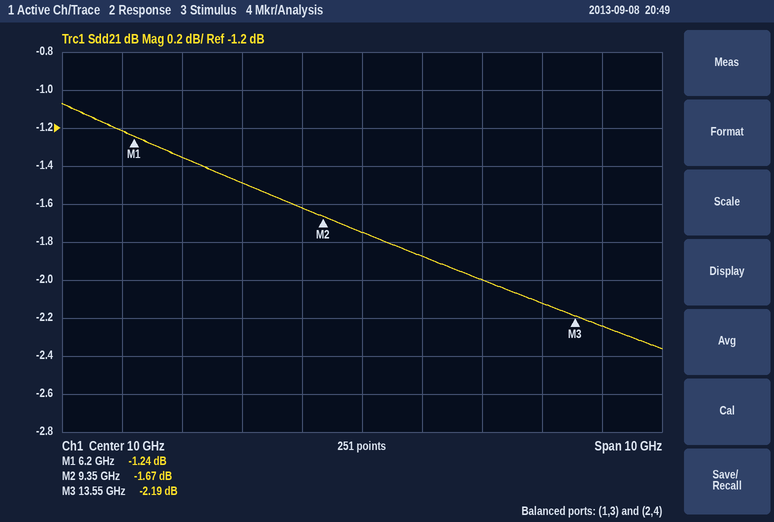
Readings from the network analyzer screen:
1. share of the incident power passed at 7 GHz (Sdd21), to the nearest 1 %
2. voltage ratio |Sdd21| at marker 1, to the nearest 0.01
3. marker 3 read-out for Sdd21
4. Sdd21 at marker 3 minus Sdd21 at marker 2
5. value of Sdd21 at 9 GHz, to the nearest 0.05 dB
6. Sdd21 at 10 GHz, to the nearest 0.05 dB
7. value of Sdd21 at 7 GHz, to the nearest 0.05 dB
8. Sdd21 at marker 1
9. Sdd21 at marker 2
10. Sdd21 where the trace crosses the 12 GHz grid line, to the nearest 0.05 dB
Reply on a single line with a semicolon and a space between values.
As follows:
73 %; 0.87; -2.19 dB; -0.52 dB; -1.60 dB; -1.75 dB; -1.35 dB; -1.24 dB; -1.67 dB; -2.00 dB
